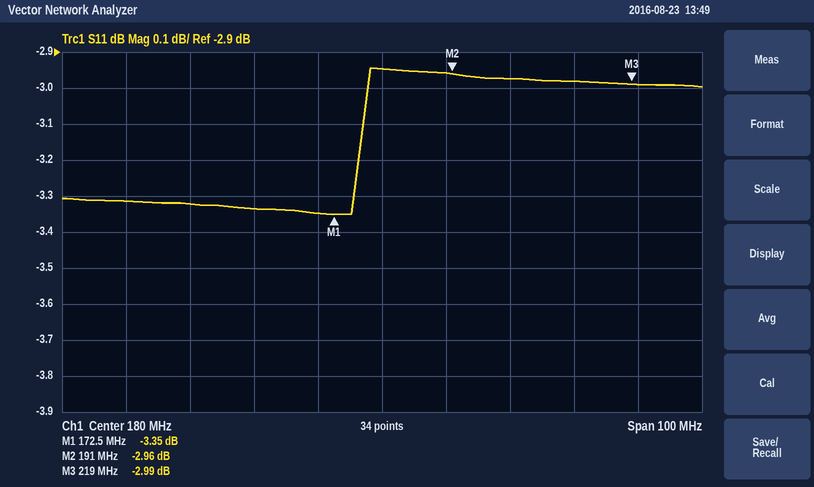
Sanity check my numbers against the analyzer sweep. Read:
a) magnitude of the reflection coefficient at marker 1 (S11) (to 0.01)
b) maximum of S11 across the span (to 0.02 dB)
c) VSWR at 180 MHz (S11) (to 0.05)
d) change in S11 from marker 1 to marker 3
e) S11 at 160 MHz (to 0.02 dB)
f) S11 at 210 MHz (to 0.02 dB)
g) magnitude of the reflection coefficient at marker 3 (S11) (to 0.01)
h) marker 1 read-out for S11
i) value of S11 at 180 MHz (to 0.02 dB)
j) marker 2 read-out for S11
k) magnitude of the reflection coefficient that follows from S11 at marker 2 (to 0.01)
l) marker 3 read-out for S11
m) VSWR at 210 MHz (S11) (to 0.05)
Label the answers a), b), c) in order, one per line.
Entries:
a) 0.68
b) -2.94 dB
c) 5.95
d) 0.36 dB
e) -3.34 dB
f) -2.98 dB
g) 0.71
h) -3.35 dB
i) -2.94 dB
j) -2.96 dB
k) 0.71
l) -2.99 dB
m) 5.90
